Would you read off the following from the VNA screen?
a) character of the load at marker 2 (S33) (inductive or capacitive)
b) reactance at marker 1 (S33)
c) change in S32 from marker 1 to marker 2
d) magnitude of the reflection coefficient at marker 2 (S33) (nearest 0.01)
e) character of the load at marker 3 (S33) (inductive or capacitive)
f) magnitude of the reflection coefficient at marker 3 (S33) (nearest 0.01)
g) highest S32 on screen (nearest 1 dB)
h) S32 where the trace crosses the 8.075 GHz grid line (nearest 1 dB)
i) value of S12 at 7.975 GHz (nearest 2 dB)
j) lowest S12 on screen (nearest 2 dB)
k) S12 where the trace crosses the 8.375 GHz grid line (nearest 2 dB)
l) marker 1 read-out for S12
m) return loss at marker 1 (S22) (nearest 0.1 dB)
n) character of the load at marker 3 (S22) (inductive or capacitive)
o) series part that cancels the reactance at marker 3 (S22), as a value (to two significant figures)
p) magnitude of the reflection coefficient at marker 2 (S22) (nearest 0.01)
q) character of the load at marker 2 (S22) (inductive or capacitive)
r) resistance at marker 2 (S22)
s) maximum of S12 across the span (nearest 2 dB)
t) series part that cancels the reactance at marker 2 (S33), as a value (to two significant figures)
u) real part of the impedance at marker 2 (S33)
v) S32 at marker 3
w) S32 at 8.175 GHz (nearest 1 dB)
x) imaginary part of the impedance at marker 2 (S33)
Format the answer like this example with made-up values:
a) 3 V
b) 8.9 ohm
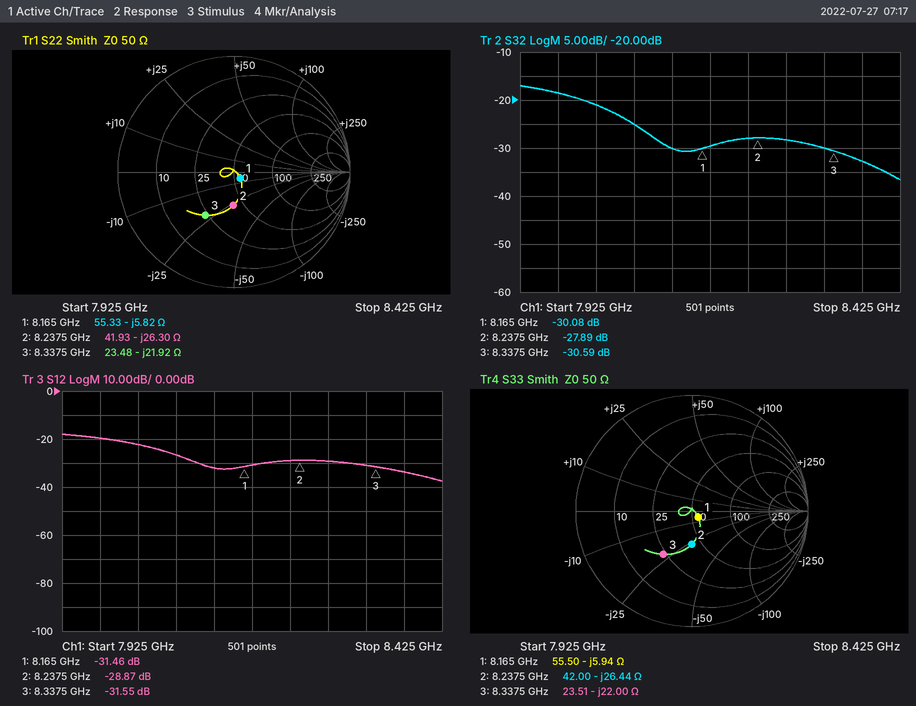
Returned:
a) capacitive
b) -5.94 Ω
c) 2.19 dB
d) 0.29
e) capacitive
f) 0.45
g) -17 dB
h) -25 dB
i) -20 dB
j) -38 dB
k) -34 dB
l) -31.46 dB
m) 22.5 dB
n) capacitive
o) 420 pH
p) 0.29
q) capacitive
r) 41.93 Ω
s) -18 dB
t) 510 pH
u) 42.00 Ω
v) -30.59 dB
w) -30 dB
x) -26.44 Ω
